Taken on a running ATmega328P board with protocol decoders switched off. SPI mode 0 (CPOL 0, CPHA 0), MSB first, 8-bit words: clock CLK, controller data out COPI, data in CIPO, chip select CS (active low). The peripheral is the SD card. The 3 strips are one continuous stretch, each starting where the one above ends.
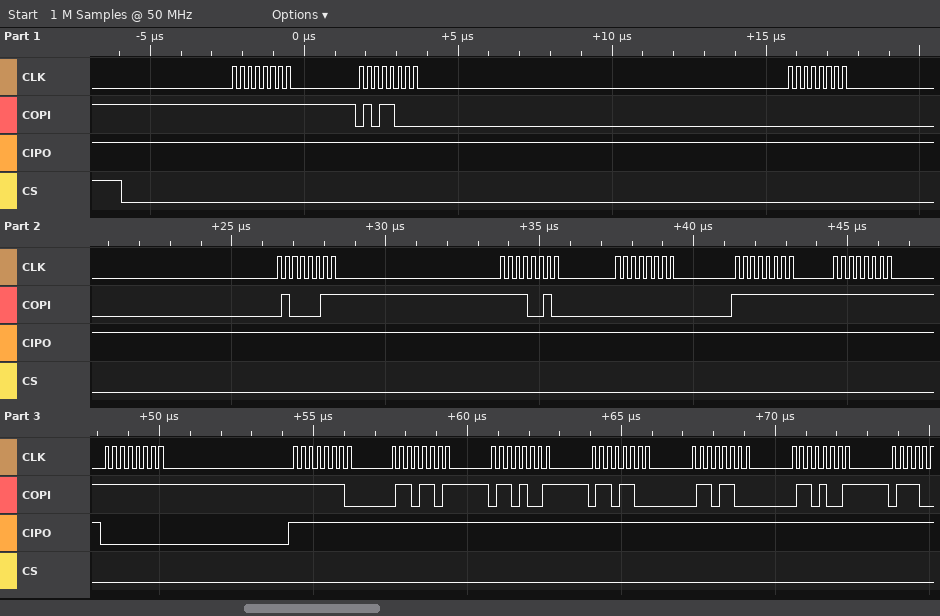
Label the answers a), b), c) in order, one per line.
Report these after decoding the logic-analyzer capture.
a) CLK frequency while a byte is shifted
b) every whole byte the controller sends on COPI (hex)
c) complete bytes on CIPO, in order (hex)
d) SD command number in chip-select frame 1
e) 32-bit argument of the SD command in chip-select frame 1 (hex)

a) 4 MHz
b) FF 58 00 43 F2 00 FF FF FF FE 6D 69 6C 6C 69
c) FF FF FF FF FF FF FF FF 00 FF FF FF FF FF FF
d) CMD24
e) 0x0043F200
